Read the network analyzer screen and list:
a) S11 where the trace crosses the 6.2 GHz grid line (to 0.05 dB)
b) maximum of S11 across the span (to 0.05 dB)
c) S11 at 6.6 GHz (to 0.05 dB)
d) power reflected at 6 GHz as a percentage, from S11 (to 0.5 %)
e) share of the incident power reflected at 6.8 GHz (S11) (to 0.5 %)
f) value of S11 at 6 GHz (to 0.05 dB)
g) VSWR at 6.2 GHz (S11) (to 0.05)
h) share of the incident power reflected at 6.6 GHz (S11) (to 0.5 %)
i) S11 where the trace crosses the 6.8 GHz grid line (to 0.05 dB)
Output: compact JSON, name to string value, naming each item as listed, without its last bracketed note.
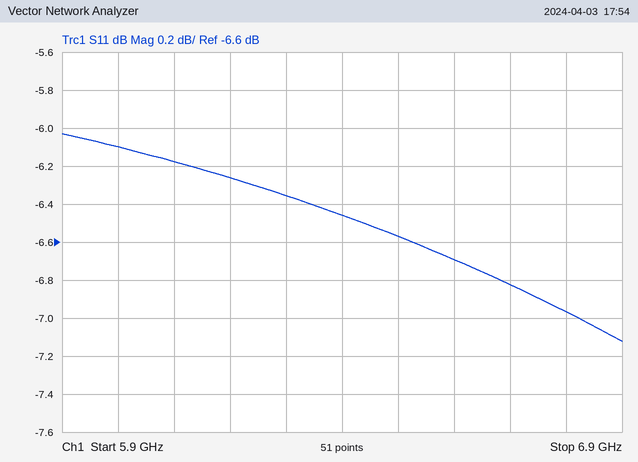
{"S11 where the trace crosses the 6.2 GHz grid line": "-6.25 dB", "maximum of S11 across the span": "-6.05 dB", "S11 at 6.6 GHz": "-6.70 dB", "power reflected at 6 GHz as a percentage, from S11": "24.5 %", "share of the incident power reflected at 6.8 GHz (S11)": "20.0 %", "value of S11 at 6 GHz": "-6.10 dB", "VSWR at 6.2 GHz (S11)": "2.90", "share of the incident power reflected at 6.6 GHz (S11)": "21.5 %", "S11 where the trace crosses the 6.8 GHz grid line": "-6.95 dB"}
